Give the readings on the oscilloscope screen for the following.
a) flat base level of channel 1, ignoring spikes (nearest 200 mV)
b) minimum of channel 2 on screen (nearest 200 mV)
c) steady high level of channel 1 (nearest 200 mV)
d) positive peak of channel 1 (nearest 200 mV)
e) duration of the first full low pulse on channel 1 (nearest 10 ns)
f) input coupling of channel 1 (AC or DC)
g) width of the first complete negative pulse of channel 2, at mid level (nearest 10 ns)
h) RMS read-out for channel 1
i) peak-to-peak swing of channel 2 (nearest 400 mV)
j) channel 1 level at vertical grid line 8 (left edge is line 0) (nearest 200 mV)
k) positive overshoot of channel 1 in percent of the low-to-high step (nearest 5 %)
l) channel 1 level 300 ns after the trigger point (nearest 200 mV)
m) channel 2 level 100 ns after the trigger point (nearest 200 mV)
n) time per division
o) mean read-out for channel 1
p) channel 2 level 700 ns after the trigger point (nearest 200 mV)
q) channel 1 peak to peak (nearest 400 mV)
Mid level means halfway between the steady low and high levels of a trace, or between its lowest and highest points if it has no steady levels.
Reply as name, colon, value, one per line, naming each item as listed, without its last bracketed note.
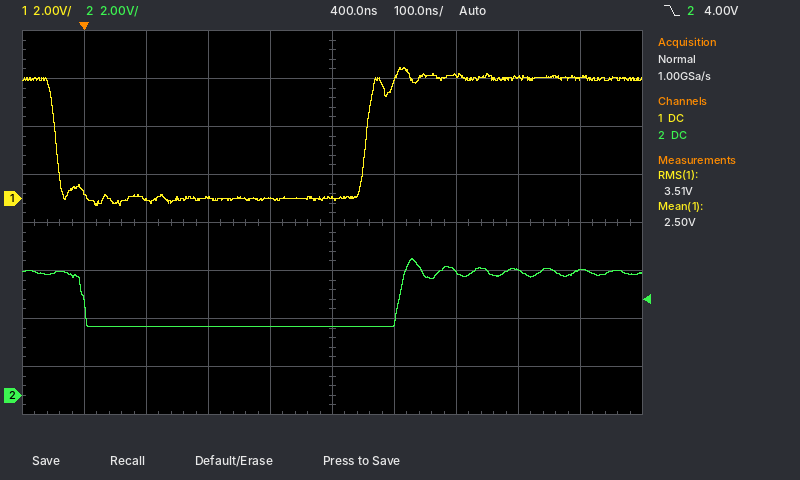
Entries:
flat base level of channel 1, ignoring spikes: 0.0 V
minimum of channel 2 on screen: 2.8 V
steady high level of channel 1: 5.0 V
positive peak of channel 1: 5.4 V
duration of the first full low pulse on channel 1: 500 ns
input coupling of channel 1: DC
width of the first complete negative pulse of channel 2, at mid level: 510 ns
RMS read-out for channel 1: 3.51 V
peak-to-peak swing of channel 2: 2.8 V
channel 1 level at vertical grid line 8 (left edge is line 0): 5.0 V
positive overshoot of channel 1 in percent of the low-to-high step: 10 %
channel 1 level 300 ns after the trigger point: 0.0 V
channel 2 level 100 ns after the trigger point: 2.8 V
time per division: 100 ns
mean read-out for channel 1: 2.50 V
channel 2 level 700 ns after the trigger point: 5.2 V
channel 1 peak to peak: 5.6 V
